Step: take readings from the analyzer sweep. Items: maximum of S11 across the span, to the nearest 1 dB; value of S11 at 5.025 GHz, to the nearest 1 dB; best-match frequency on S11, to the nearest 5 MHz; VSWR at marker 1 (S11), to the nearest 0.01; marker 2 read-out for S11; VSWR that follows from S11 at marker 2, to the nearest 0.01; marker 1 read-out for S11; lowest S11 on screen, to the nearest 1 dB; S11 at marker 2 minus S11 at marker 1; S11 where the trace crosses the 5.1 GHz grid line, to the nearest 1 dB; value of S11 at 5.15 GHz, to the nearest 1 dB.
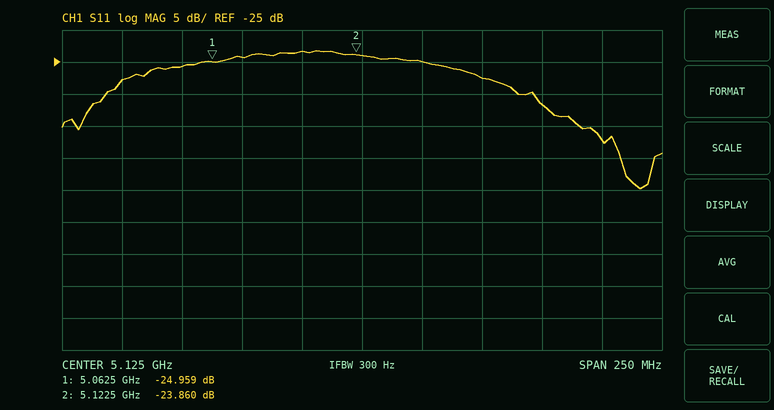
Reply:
-23 dB
-28 dB
5.240 GHz
1.12
-23.860 dB
1.14
-24.959 dB
-45 dB
1.099 dB
-23 dB
-25 dB
